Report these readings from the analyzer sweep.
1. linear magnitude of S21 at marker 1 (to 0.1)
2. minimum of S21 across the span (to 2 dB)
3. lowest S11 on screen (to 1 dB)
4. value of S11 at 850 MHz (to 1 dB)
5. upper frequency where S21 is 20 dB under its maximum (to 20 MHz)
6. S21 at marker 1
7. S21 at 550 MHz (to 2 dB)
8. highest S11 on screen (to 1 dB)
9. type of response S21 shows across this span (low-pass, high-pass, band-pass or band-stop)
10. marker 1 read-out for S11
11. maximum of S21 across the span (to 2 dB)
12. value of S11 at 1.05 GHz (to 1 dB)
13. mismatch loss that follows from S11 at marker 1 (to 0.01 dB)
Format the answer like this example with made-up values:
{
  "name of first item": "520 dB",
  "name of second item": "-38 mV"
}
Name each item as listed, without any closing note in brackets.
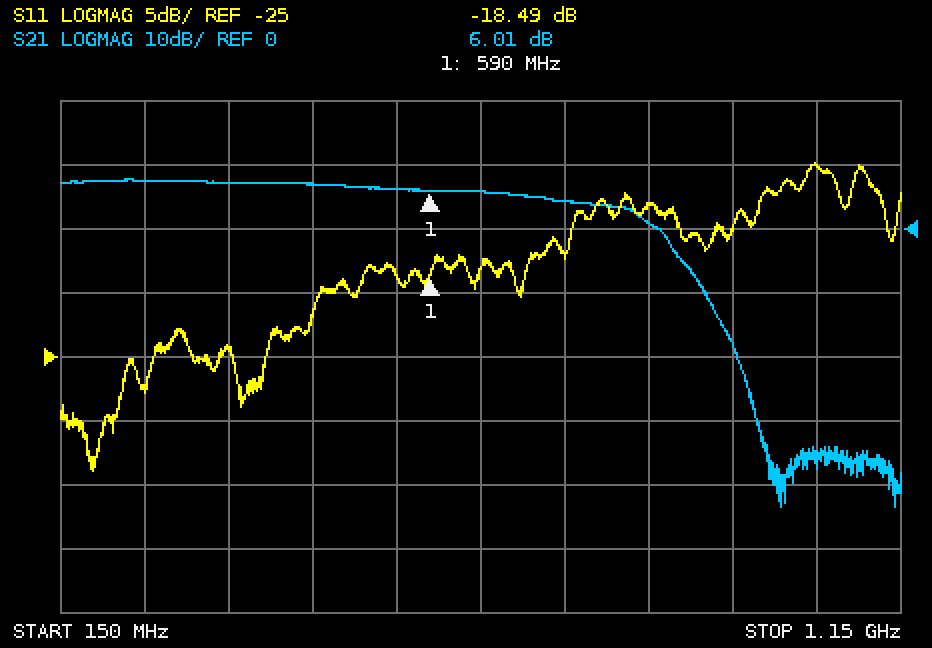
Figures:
{
  "linear magnitude of S21 at marker 1": "2.0",
  "minimum of S21 across the span": "-44 dB",
  "lowest S11 on screen": "-34 dB",
  "value of S11 at 850 MHz": "-13 dB",
  "upper frequency where S21 is 20 dB under its maximum": "920 MHz",
  "S21 at marker 1": "6.01 dB",
  "S21 at 550 MHz": "6 dB",
  "highest S11 on screen": "-10 dB",
  "type of response S21 shows across this span": "low-pass",
  "marker 1 read-out for S11": "-18.49 dB",
  "maximum of S21 across the span": "8 dB",
  "value of S11 at 1.05 GHz": "-10 dB",
  "mismatch loss that follows from S11 at marker 1": "0.06 dB"
}
